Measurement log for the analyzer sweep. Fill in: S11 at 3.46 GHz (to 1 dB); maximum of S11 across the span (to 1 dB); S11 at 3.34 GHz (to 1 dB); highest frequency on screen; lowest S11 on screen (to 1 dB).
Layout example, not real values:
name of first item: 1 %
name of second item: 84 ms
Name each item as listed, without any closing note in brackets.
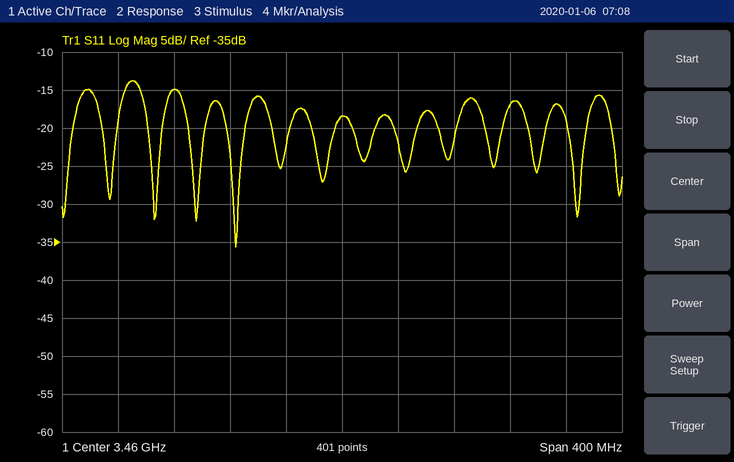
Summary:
S11 at 3.46 GHz: -18 dB
maximum of S11 across the span: -14 dB
S11 at 3.34 GHz: -15 dB
highest frequency on screen: 3.66 GHz
lowest S11 on screen: -36 dB
